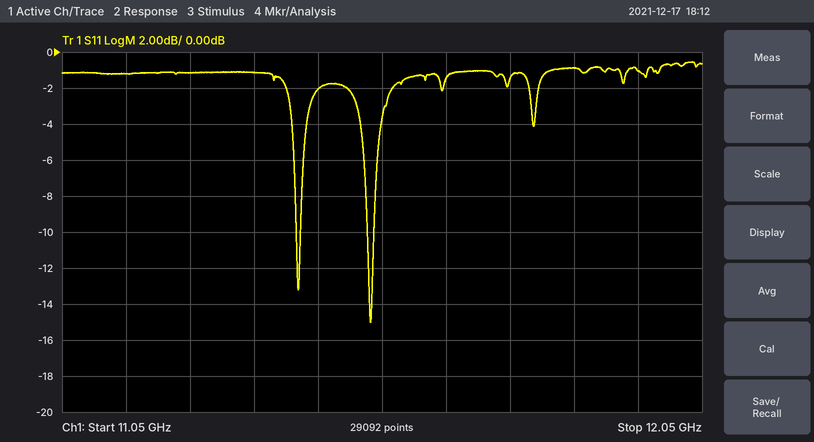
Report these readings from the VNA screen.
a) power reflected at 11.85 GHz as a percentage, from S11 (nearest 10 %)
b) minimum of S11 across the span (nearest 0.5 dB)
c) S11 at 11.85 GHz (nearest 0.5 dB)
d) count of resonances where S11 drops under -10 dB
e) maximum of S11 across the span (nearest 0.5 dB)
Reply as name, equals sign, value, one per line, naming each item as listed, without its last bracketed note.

power reflected at 11.85 GHz as a percentage, from S11 = 80 %
minimum of S11 across the span = -15.0 dB
S11 at 11.85 GHz = -1.0 dB
count of resonances where S11 drops under -10 dB = 2
maximum of S11 across the span = -0.5 dB
